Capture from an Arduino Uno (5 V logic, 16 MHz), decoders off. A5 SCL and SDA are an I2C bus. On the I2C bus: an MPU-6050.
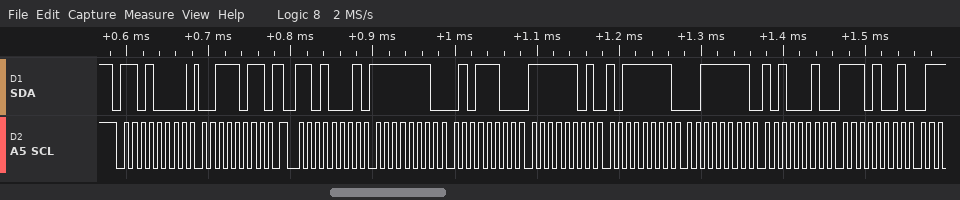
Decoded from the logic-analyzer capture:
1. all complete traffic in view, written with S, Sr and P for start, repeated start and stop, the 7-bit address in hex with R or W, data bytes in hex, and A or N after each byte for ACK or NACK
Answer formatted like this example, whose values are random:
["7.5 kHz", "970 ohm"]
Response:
["S 68W A 3B A Sr 68R A FE A 5C A FD A BF A 3F A A2 A E9 A"]
